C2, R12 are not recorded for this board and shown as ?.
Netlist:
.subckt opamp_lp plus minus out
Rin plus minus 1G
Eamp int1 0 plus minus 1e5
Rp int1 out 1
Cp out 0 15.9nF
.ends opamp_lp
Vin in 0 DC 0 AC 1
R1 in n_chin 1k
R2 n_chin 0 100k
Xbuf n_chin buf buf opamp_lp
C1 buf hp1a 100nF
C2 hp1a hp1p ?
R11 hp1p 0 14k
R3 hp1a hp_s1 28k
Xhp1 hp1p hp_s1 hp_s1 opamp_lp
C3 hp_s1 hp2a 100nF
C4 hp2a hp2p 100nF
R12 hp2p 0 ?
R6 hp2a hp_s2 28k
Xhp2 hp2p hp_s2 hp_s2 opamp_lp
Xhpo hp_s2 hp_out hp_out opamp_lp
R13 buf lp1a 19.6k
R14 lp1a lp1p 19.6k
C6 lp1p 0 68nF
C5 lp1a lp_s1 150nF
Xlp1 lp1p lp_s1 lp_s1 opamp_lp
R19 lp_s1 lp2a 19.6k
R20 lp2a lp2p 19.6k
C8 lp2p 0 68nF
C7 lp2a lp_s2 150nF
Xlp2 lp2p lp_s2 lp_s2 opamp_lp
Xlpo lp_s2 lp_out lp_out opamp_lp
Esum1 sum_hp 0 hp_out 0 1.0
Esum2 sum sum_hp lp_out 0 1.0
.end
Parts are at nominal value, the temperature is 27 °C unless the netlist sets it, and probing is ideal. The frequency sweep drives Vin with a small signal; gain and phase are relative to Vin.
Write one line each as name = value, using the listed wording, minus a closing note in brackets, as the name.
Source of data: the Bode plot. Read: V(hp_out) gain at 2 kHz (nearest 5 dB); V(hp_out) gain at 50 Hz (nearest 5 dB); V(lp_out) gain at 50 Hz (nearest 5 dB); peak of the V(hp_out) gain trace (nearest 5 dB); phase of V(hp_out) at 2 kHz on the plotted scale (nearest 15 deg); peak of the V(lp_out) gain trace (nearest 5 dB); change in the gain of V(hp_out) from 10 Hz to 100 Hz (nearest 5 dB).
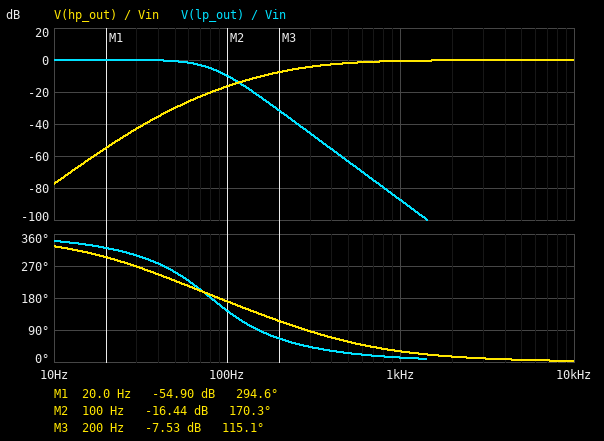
V(hp_out) gain at 2 kHz = 0 dB
V(hp_out) gain at 50 Hz = -30 dB
V(lp_out) gain at 50 Hz = 0 dB
peak of the V(hp_out) gain trace = 0 dB
phase of V(hp_out) at 2 kHz on the plotted scale = 15 deg
peak of the V(lp_out) gain trace = 0 dB
change in the gain of V(hp_out) from 10 Hz to 100 Hz = 60 dB
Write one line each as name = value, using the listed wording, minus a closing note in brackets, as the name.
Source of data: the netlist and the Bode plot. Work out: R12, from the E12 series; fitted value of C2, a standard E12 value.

R12, from the E12 series = 18 kΩ
fitted value of C2, a standard E12 value = 47 nF
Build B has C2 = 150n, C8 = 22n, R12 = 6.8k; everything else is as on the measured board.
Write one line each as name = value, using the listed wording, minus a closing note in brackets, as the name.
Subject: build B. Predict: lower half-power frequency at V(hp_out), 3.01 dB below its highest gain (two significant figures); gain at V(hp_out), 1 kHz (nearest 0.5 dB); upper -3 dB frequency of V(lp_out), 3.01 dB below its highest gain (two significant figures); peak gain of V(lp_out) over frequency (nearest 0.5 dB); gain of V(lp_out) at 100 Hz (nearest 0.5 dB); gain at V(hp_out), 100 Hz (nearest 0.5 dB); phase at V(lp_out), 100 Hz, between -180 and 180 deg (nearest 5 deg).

lower half-power frequency at V(hp_out), 3.01 dB below its highest gain = 490 Hz
gain at V(hp_out), 1 kHz = -1.0 dB
upper -3 dB frequency of V(lp_out), 3.01 dB below its highest gain = 100 Hz
peak gain of V(lp_out) over frequency = 0.5 dB
gain of V(lp_out) at 100 Hz = -2.5 dB
gain at V(hp_out), 100 Hz = -19.5 dB
phase at V(lp_out), 100 Hz, between -180 and 180 deg = -155 deg
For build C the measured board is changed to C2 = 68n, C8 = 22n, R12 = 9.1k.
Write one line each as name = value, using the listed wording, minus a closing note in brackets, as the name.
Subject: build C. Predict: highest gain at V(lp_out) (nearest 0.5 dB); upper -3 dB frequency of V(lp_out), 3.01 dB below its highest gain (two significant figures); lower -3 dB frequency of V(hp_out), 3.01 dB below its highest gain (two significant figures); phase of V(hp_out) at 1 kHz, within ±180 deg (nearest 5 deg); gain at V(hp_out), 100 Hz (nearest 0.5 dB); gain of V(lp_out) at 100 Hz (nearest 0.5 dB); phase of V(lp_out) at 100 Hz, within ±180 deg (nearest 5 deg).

highest gain at V(lp_out) = 0.5 dB
upper -3 dB frequency of V(lp_out), 3.01 dB below its highest gain = 100 Hz
lower -3 dB frequency of V(hp_out), 3.01 dB below its highest gain = 440 Hz
phase of V(hp_out) at 1 kHz, within ±180 deg = 35 deg
gain at V(hp_out), 100 Hz = -20.0 dB
gain of V(lp_out) at 100 Hz = -2.5 dB
phase of V(lp_out) at 100 Hz, within ±180 deg = -155 deg
